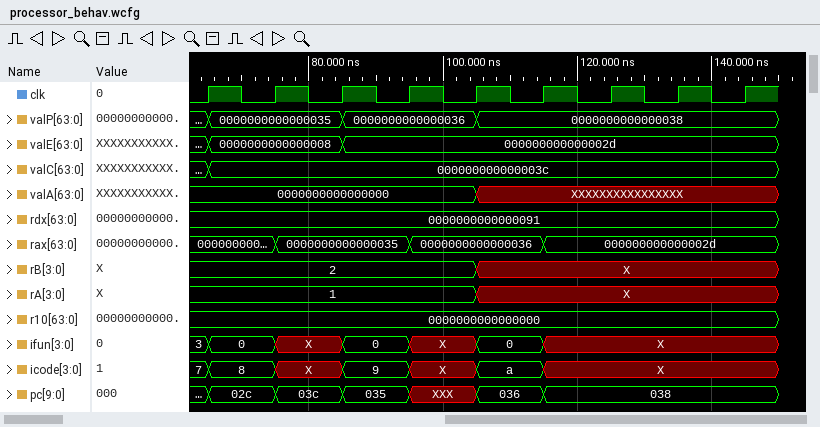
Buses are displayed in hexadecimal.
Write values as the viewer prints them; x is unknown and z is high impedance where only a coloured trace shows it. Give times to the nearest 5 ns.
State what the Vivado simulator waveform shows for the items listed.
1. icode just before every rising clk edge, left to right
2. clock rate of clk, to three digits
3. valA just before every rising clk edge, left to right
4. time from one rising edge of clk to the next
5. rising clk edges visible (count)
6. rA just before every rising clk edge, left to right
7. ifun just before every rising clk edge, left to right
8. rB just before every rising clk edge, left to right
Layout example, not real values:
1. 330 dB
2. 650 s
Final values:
1. 7, 8, X, 9, X, a, X, X, X
2. 100 MHz
3. 0000000000000000, 0000000000000000, 0000000000000000, 0000000000000000, 0000000000000000, XXXXXXXXXXXXXXXX, XXXXXXXXXXXXXXXX, XXXXXXXXXXXXXXXX, XXXXXXXXXXXXXXXX
4. 10 ns
5. 9
6. 1, 1, 1, 1, 1, X, X, X, X
7. 3, 0, X, 0, X, 0, X, X, X
8. 2, 2, 2, 2, 2, X, X, X, X
